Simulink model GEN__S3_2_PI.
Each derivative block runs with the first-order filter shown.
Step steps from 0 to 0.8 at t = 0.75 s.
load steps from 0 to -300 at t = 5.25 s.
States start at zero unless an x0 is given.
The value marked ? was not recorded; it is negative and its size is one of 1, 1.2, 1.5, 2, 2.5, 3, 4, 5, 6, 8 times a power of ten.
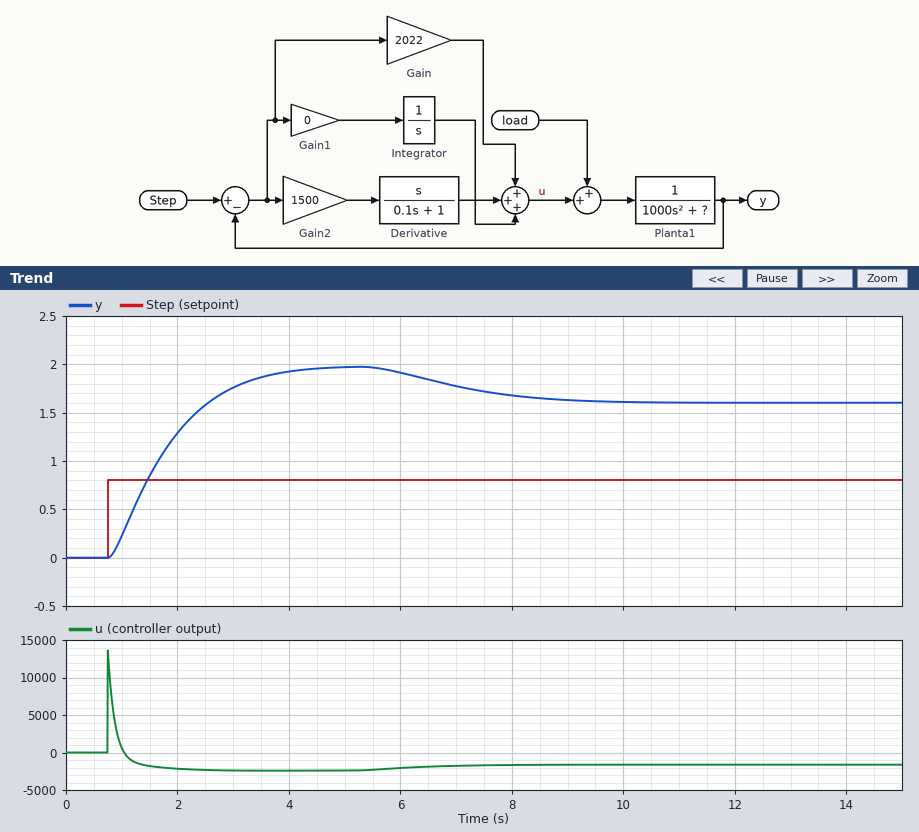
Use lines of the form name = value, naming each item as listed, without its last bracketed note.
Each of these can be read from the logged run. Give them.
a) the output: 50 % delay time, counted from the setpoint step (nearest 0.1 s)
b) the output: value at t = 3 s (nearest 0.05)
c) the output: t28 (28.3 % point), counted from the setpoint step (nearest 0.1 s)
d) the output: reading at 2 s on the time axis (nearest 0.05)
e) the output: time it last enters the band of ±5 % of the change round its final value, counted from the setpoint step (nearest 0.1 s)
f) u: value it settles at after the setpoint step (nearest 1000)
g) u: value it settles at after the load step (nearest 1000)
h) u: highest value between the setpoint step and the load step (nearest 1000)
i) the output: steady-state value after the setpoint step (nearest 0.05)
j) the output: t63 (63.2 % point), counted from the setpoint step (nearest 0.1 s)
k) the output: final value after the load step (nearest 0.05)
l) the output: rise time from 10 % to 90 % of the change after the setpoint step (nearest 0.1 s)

the output: 50 % delay time, counted from the setpoint step = 0.9 s
the output: value at t = 3 s = 1.75
the output: t28 (28.3 % point), counted from the setpoint step = 0.5 s
the output: reading at 2 s on the time axis = 1.30
the output: time it last enters the band of ±5 % of the change round its final value, counted from the setpoint step = 2.8 s
u: value it settles at after the setpoint step = -2000
u: value it settles at after the load step = -2000
u: highest value between the setpoint step and the load step = 14000
the output: steady-state value after the setpoint step = 1.95
the output: t63 (63.2 % point), counted from the setpoint step = 1.2 s
the output: final value after the load step = 1.60
the output: rise time from 10 % to 90 % of the change after the setpoint step = 2.1 s
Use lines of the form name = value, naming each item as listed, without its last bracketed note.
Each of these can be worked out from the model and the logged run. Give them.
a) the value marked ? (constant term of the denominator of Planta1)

the value marked ? = -1200
